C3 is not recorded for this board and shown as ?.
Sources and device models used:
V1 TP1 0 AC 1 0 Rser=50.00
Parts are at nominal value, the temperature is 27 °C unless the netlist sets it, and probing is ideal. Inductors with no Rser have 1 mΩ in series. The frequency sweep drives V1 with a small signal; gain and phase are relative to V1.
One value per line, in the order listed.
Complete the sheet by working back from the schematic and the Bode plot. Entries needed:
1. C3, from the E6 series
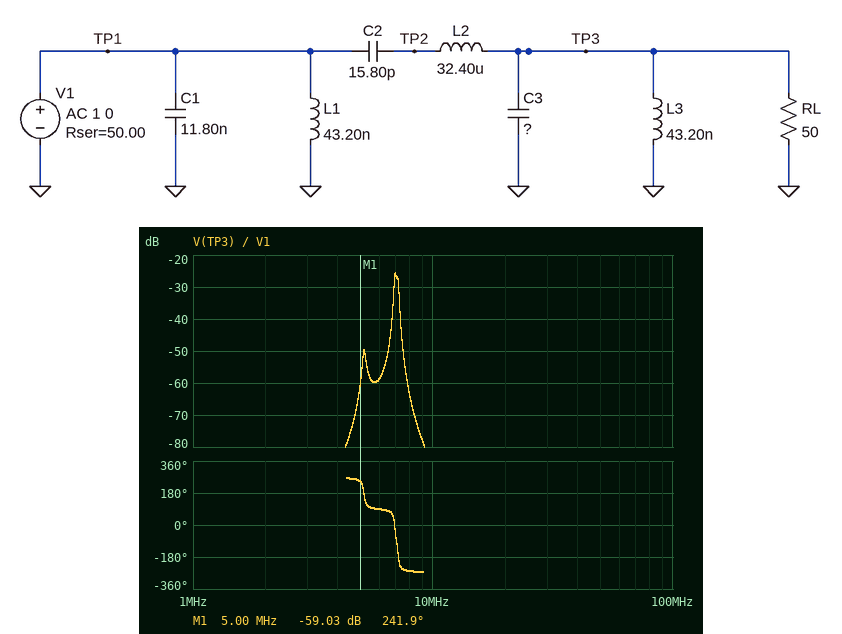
22 nF
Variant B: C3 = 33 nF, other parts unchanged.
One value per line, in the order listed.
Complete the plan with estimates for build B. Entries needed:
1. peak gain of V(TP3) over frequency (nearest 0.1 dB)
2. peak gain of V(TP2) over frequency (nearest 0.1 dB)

-31.9 dB
30.3 dB
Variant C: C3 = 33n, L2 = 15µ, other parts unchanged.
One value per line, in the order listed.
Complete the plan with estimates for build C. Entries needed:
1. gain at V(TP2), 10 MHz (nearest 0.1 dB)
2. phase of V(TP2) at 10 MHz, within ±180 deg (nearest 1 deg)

-2.6 dB
93 deg
